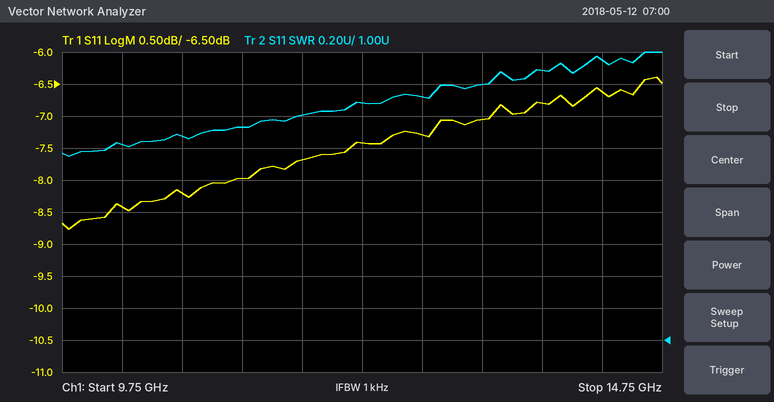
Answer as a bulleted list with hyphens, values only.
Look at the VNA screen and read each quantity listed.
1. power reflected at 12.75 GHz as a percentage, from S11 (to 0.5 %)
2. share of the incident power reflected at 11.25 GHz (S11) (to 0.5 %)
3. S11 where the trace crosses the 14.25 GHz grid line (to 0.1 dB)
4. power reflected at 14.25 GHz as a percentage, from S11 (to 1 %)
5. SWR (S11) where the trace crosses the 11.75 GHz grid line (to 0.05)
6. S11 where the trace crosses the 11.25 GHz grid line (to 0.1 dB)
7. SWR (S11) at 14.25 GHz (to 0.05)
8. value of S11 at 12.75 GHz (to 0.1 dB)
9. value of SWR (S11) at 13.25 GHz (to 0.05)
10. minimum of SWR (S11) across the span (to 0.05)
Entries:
- 18.5 %
- 16.0 %
- -6.6 dB
- 22 %
- 2.40
- -8.0 dB
- 2.75
- -7.3 dB
- 2.60
- 2.15
